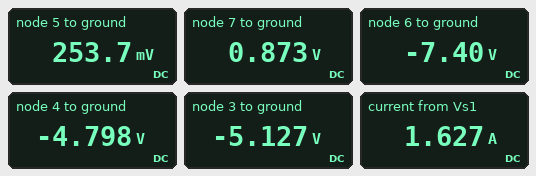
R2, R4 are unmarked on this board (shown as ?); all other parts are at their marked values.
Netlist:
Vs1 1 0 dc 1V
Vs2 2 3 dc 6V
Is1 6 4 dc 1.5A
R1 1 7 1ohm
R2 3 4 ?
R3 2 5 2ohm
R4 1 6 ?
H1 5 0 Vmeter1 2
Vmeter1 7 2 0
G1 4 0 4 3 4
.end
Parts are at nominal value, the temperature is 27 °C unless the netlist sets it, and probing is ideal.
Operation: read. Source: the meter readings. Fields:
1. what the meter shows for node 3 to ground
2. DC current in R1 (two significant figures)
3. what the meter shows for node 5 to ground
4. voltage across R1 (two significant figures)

-5.127 V
130 mA
253.7 mV
130 mV
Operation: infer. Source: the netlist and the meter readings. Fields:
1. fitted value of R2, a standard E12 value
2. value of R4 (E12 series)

1.8 Ω
5.6 Ω
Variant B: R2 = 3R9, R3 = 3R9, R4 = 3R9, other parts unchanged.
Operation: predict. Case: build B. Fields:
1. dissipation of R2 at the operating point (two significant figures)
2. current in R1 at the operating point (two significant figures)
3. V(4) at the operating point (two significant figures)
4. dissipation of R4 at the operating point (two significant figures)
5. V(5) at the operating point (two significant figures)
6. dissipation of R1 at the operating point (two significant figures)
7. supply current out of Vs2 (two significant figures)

32 mW
94 mA
-4.7 V
8.8 W
190 mV
8.8 mW
90 mA
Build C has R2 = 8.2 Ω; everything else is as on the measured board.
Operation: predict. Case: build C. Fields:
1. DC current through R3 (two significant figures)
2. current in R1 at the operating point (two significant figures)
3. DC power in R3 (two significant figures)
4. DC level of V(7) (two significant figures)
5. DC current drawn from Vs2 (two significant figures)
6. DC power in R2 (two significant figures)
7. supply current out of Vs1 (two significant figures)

230 mA
180 mA
100 mW
820 mV
44 mA
16 mW
1.7 A
